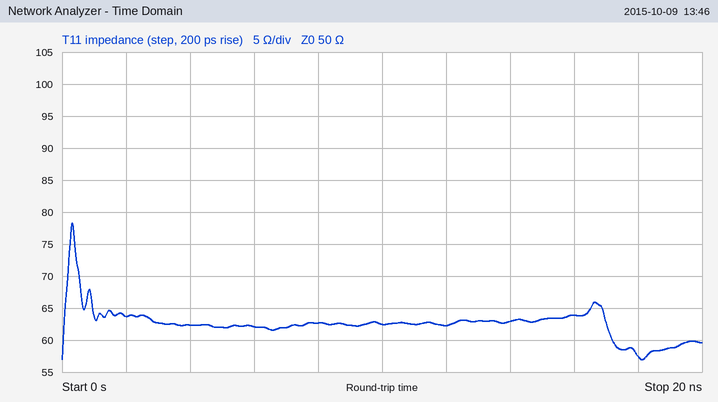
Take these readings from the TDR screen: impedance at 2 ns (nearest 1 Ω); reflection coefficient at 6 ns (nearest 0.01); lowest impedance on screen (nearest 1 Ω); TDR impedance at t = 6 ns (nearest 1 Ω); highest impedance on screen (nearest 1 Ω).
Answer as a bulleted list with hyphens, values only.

- 64 Ω
- +0.11
- 57 Ω
- 62 Ω
- 78 Ω
